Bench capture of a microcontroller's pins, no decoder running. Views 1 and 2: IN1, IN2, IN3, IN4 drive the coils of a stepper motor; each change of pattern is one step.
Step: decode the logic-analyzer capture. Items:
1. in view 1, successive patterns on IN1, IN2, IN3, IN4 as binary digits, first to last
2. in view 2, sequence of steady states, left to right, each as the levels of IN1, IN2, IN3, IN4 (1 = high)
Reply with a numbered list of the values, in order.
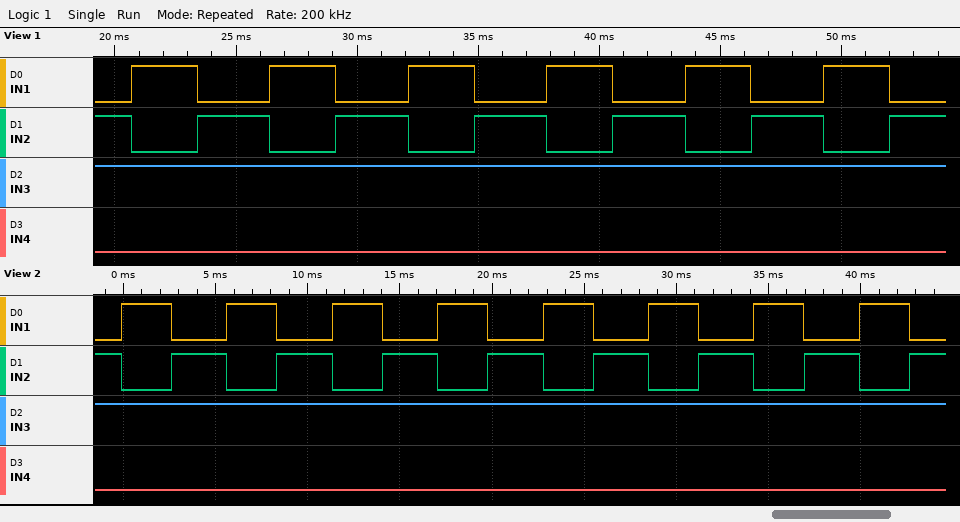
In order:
1. 0110 1010 0110 1010 0110 1010 0110 1010 0110 1010 0110 1010 0110
2. 0110 1010 0110 1010 0110 1010 0110 1010 0110 1010 0110 1010 0110 1010 0110 1010 0110
